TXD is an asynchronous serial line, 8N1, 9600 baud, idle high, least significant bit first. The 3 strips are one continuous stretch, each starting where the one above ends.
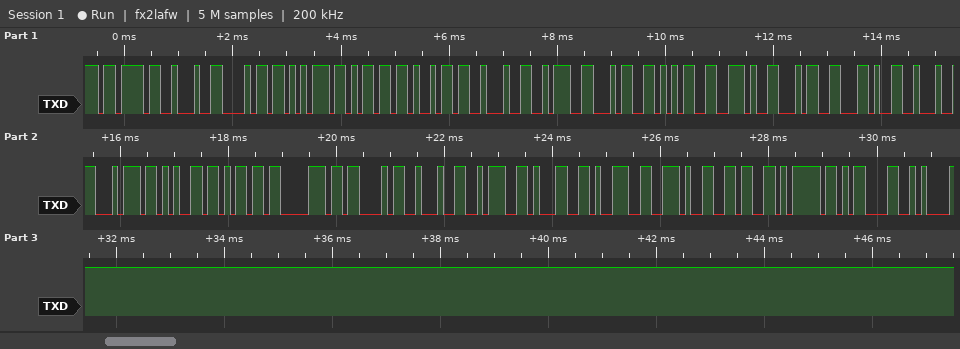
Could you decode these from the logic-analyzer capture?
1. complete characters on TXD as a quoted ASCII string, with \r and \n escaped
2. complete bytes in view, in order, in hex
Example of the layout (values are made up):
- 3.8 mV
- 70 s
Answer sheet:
- "{\"humi\":45.4,\"tempC\":19.6}\r\n"
- 7B 22 68 75 6D 69 22 3A 34 35 2E 34 2C 22 74 65 6D 70 43 22 3A 31 39 2E 36 7D 0D 0A
